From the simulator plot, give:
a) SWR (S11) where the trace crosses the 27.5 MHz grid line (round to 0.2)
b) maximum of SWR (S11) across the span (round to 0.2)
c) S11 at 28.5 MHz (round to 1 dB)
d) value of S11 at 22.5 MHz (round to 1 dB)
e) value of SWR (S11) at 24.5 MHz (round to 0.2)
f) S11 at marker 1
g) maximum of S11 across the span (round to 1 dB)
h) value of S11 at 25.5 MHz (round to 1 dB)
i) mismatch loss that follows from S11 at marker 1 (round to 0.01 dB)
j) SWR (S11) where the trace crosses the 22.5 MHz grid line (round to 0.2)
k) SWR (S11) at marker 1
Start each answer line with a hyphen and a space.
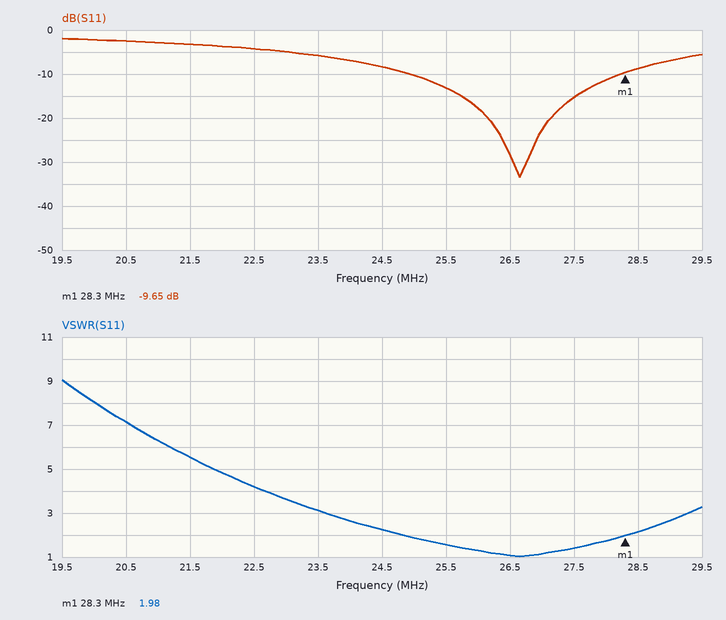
- 1.4
- 9.0
- -9 dB
- -4 dB
- 2.2
- -9.65 dB
- -2 dB
- -13 dB
- 0.50 dB
- 4.2
- 1.98
